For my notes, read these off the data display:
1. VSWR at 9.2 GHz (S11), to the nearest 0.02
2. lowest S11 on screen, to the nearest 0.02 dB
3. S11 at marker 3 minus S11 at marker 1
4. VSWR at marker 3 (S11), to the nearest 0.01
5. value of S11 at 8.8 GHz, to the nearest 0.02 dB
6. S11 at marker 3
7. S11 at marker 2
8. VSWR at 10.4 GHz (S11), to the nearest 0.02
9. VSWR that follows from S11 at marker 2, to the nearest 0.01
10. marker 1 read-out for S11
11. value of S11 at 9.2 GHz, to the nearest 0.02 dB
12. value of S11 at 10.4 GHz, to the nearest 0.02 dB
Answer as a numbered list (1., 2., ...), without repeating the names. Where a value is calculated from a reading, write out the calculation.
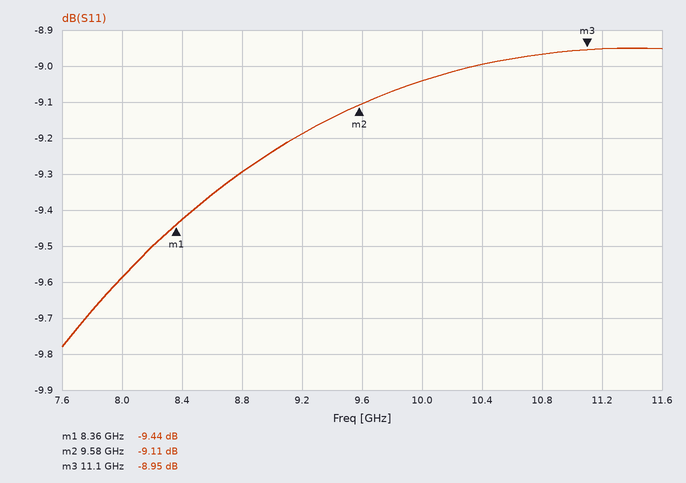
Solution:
1. |Γ| = 10^(-9.18/20) = 0.3475; VSWR = (1 + 0.3475)/(1 − 0.3475) ≈ 2.07, so 2.06 to the nearest 0.02
2. -9.78 dB
3. -8.95 − (-9.44) = 0.49 dB
4. (1 + 0.3569)/(1 − 0.3569) ≈ 2.11
5. -9.30 dB
6. -8.95 dB
7. -9.11 dB
8. |Γ| = 10^(-9/20) = 0.3548; VSWR = (1 + 0.3548)/(1 − 0.3548) ≈ 2.10
9. (1 + 0.3503)/(1 − 0.3503) ≈ 2.08
10. -9.44 dB
11. -9.18 dB
12. -9.00 dB
